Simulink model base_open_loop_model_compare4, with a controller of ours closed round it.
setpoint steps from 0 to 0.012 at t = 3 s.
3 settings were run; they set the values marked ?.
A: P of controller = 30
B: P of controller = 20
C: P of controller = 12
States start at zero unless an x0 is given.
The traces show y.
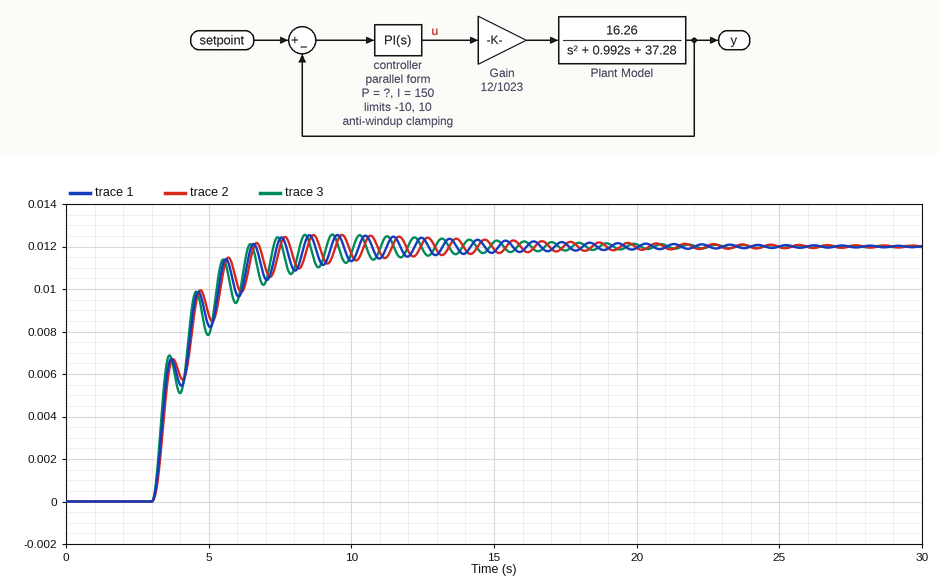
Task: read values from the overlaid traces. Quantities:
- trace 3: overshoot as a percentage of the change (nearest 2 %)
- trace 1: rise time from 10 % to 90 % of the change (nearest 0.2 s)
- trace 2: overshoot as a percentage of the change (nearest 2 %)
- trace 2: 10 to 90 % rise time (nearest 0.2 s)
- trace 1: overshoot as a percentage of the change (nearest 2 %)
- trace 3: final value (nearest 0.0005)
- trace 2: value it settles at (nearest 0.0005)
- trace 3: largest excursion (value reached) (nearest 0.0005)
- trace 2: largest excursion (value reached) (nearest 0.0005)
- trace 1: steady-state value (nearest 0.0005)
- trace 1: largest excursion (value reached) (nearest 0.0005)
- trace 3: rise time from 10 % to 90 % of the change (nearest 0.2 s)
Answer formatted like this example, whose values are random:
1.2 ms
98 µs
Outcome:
4 %
2.2 s
4 %
2.2 s
4 %
0.0120
0.0120
0.0125
0.0125
0.0120
0.0125
2.2 s
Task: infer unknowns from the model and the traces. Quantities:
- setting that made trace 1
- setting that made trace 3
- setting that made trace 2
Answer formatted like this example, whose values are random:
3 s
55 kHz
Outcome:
B
A
C
